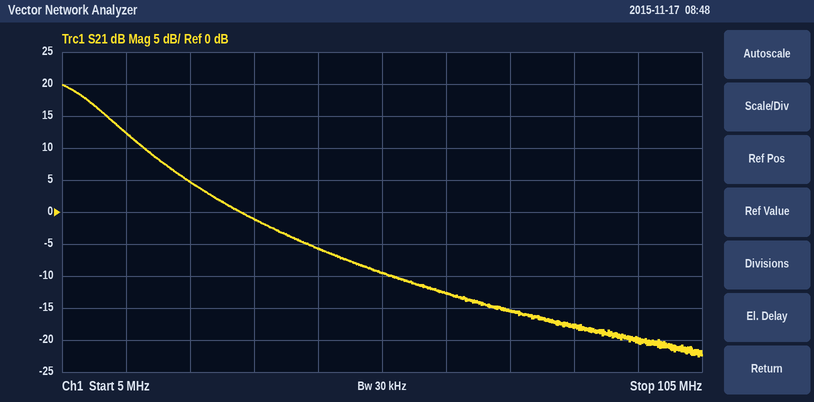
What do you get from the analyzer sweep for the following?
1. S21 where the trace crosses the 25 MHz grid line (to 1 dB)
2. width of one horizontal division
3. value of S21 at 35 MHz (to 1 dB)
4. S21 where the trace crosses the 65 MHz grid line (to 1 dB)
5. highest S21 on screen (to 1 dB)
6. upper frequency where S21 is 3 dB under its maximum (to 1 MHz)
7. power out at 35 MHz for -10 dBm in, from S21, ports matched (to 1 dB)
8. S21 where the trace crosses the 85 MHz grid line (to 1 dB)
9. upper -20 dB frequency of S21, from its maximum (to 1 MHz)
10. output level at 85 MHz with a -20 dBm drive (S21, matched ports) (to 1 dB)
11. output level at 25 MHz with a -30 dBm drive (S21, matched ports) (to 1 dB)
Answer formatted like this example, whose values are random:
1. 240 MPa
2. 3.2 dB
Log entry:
1. 5 dB
2. 10 MHz
3. -1 dB
4. -13 dB
5. 20 dB
6. 10 MHz
7. -11 dBm
8. -18 dB
9. 33 MHz
10. -38 dBm
11. -25 dBm
